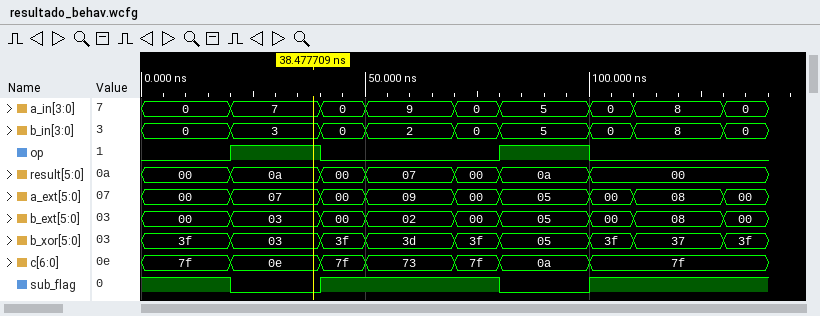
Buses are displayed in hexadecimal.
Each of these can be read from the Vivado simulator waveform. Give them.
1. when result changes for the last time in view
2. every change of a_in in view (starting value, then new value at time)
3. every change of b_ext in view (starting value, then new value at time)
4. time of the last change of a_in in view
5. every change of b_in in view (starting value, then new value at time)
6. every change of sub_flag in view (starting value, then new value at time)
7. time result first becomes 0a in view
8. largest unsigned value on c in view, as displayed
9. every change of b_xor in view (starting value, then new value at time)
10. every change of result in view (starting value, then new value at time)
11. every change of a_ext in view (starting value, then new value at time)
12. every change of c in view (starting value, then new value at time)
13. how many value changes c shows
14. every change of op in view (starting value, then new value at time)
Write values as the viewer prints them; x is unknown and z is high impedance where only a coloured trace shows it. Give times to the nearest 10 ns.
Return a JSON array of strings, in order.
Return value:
["100 ns", "0, 7 at 20 ns, 0 at 40 ns, 9 at 50 ns, 0 at 70 ns, 5 at 80 ns, 0 at 100 ns, 8 at 110 ns, 0 at 130 ns", "00, 03 at 20 ns, 00 at 40 ns, 02 at 50 ns, 00 at 70 ns, 05 at 80 ns, 00 at 100 ns, 08 at 110 ns, 00 at 130 ns", "130 ns", "0, 3 at 20 ns, 0 at 40 ns, 2 at 50 ns, 0 at 70 ns, 5 at 80 ns, 0 at 100 ns, 8 at 110 ns, 0 at 130 ns", "1, 0 at 20 ns, 1 at 40 ns, 0 at 80 ns, 1 at 100 ns", "20 ns", "7f", "3f, 03 at 20 ns, 3f at 40 ns, 3d at 50 ns, 3f at 70 ns, 05 at 80 ns, 3f at 100 ns, 37 at 110 ns, 3f at 130 ns", "00, 0a at 20 ns, 00 at 40 ns, 07 at 50 ns, 00 at 70 ns, 0a at 80 ns, 00 at 100 ns", "00, 07 at 20 ns, 00 at 40 ns, 09 at 50 ns, 00 at 70 ns, 05 at 80 ns, 00 at 100 ns, 08 at 110 ns, 00 at 130 ns", "7f, 0e at 20 ns, 7f at 40 ns, 73 at 50 ns, 7f at 70 ns, 0a at 80 ns, 7f at 100 ns", "6", "0, 1 at 20 ns, 0 at 40 ns, 1 at 80 ns, 0 at 100 ns"]
